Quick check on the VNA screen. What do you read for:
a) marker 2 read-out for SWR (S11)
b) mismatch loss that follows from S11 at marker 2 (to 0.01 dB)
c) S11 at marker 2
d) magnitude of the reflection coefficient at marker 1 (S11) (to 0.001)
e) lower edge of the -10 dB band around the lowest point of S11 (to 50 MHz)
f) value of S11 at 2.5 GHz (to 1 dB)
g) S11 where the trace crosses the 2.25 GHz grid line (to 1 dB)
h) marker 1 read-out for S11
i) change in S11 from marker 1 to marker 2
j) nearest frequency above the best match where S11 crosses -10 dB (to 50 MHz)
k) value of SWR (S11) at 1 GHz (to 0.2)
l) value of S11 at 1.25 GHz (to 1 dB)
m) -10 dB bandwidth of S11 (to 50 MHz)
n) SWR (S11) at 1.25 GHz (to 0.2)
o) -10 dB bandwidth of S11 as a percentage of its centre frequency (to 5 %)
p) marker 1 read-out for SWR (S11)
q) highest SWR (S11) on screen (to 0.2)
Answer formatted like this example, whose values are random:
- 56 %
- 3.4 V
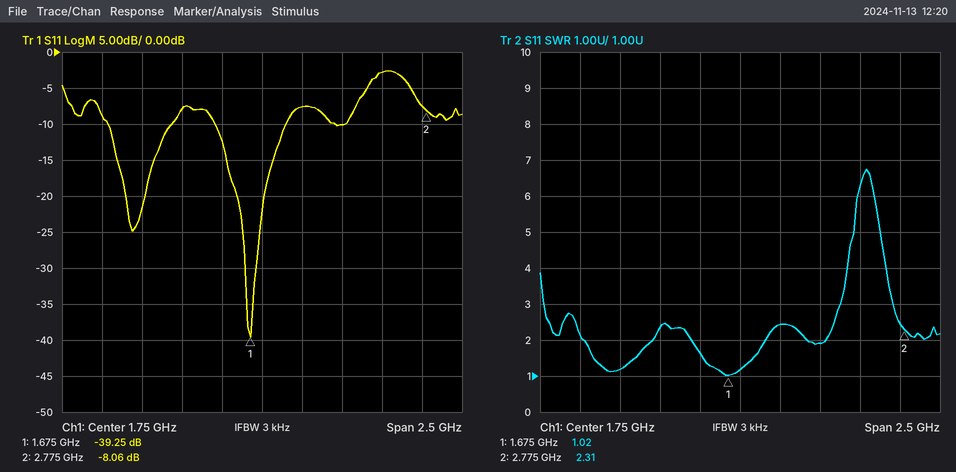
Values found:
- 2.31
- 0.74 dB
- -8.06 dB
- 0.011
- 1.45 GHz
- -3 dB
- -10 dB
- -39.25 dB
- 31.19 dB
- 1.90 GHz
- 1.2
- -8 dB
- 450 MHz
- 2.4
- 25 %
- 1.02
- 6.8
